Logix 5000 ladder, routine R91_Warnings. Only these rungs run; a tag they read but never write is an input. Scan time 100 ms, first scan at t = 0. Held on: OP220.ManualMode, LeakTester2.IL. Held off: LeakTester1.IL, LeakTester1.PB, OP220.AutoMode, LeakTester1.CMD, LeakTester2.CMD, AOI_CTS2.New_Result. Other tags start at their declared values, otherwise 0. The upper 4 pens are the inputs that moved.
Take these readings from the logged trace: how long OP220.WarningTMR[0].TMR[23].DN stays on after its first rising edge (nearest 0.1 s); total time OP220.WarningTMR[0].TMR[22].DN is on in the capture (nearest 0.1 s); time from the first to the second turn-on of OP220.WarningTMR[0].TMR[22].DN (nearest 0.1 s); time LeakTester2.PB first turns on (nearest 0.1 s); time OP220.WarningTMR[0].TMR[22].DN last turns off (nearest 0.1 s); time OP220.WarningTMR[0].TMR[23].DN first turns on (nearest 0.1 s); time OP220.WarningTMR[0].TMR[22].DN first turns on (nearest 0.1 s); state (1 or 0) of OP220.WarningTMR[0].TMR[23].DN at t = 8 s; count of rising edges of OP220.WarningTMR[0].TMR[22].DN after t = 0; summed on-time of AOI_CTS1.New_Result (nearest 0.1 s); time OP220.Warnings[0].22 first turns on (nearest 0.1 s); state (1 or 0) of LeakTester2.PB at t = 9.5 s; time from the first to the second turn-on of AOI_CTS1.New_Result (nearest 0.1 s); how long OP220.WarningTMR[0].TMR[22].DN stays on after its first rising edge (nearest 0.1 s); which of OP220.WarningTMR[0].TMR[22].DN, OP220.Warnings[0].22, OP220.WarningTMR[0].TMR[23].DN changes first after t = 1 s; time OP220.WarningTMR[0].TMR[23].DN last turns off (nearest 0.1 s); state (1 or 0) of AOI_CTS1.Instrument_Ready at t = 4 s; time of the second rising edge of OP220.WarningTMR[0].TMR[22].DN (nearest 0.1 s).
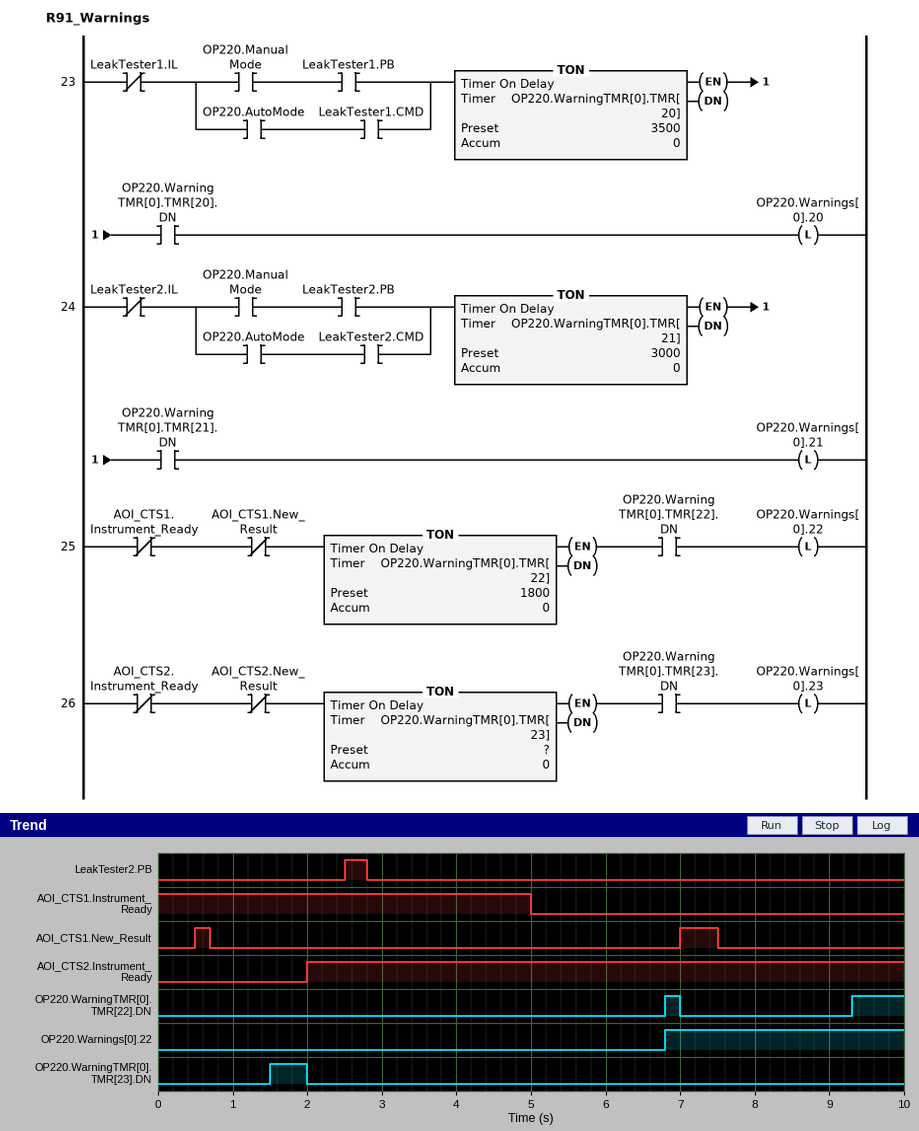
0.5 s
0.9 s
2.5 s
2.5 s
7.0 s
1.5 s
6.8 s
0
2
0.7 s
6.8 s
0
6.5 s
0.2 s
OP220.WarningTMR[0].TMR[23].DN
2.0 s
1
9.3 s
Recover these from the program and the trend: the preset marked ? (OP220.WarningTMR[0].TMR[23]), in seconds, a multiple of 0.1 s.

1.5 s
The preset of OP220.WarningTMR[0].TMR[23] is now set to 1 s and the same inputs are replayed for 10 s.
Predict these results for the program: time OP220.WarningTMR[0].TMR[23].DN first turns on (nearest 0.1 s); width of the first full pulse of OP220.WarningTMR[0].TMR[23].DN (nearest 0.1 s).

1.0 s
1.0 s
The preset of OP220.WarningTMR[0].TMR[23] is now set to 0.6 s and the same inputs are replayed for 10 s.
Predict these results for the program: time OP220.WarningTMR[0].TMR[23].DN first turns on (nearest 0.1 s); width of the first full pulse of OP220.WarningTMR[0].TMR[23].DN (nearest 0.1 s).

0.6 s
1.4 s
